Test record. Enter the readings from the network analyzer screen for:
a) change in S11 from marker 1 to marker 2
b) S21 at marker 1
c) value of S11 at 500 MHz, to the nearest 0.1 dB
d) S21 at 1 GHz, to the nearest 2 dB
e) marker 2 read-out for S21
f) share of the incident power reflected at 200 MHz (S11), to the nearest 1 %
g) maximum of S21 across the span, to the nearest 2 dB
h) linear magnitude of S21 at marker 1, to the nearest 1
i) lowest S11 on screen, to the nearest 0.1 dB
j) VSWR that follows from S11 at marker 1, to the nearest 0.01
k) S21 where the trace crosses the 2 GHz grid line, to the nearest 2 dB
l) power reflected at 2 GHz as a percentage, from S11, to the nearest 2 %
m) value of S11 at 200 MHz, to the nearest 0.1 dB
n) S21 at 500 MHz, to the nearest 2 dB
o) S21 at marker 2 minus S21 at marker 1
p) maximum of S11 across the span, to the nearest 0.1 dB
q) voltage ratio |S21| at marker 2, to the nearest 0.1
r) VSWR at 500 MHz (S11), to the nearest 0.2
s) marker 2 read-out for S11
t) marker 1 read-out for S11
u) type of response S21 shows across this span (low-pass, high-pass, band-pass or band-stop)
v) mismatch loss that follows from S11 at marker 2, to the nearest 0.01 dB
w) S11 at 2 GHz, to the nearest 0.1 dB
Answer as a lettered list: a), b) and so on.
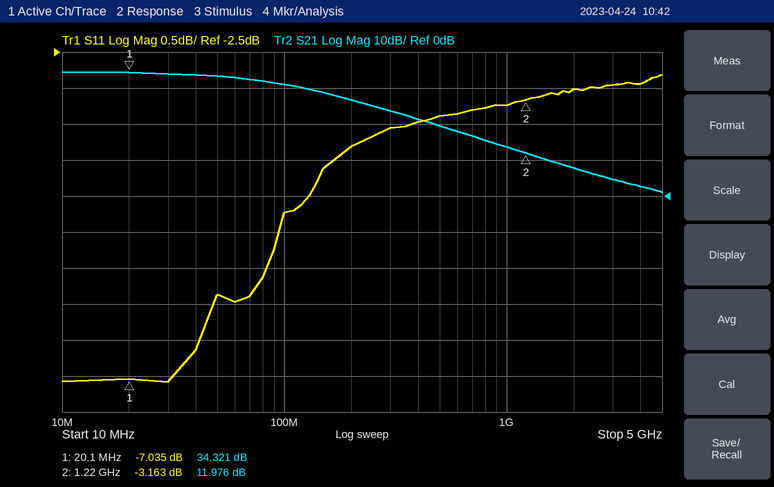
a) 3.872 dB
b) 34.321 dB
c) -3.4 dB
d) 14 dB
e) 11.976 dB
f) 42 %
g) 34 dB
h) 52
i) -7.1 dB
j) 2.60
k) 8 dB
l) 50 %
m) -3.8 dB
n) 20 dB
o) -22.345 dB
p) -2.8 dB
q) 4.0
r) 5.2
s) -3.163 dB
t) -7.035 dB
u) low-pass
v) 2.86 dB
w) -3.0 dB
